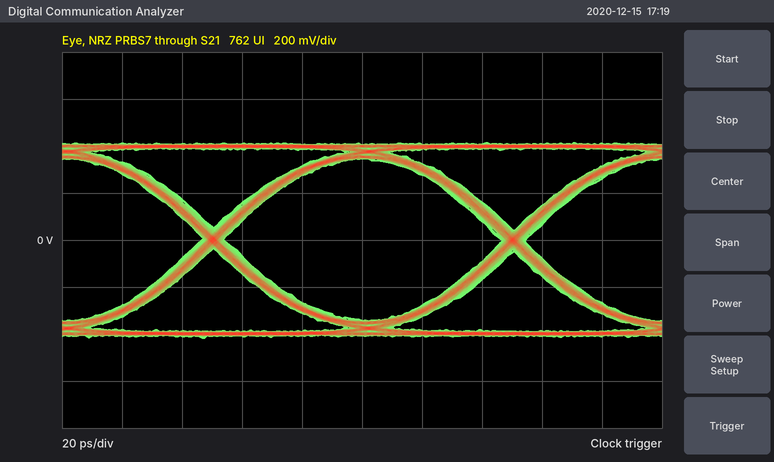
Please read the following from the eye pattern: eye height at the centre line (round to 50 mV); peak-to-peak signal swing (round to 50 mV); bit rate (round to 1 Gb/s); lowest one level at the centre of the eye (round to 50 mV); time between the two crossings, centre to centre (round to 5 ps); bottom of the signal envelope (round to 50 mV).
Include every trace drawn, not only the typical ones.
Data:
700 mV
850 mV
10 Gb/s
350 mV
100 ps
-400 mV
